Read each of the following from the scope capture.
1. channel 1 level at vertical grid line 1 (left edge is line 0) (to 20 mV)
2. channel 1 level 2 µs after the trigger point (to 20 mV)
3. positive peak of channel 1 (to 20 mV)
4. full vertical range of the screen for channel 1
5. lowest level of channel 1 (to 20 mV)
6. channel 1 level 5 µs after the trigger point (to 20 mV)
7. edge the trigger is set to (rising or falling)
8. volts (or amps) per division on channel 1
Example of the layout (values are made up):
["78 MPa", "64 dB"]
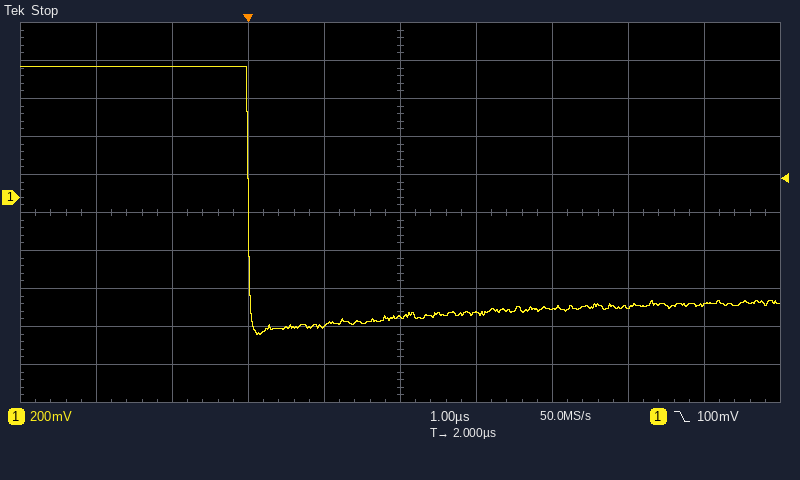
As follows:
["680 mV", "-640 mV", "680 mV", "2 V", "-720 mV", "-580 mV", "falling", "200 mV"]
